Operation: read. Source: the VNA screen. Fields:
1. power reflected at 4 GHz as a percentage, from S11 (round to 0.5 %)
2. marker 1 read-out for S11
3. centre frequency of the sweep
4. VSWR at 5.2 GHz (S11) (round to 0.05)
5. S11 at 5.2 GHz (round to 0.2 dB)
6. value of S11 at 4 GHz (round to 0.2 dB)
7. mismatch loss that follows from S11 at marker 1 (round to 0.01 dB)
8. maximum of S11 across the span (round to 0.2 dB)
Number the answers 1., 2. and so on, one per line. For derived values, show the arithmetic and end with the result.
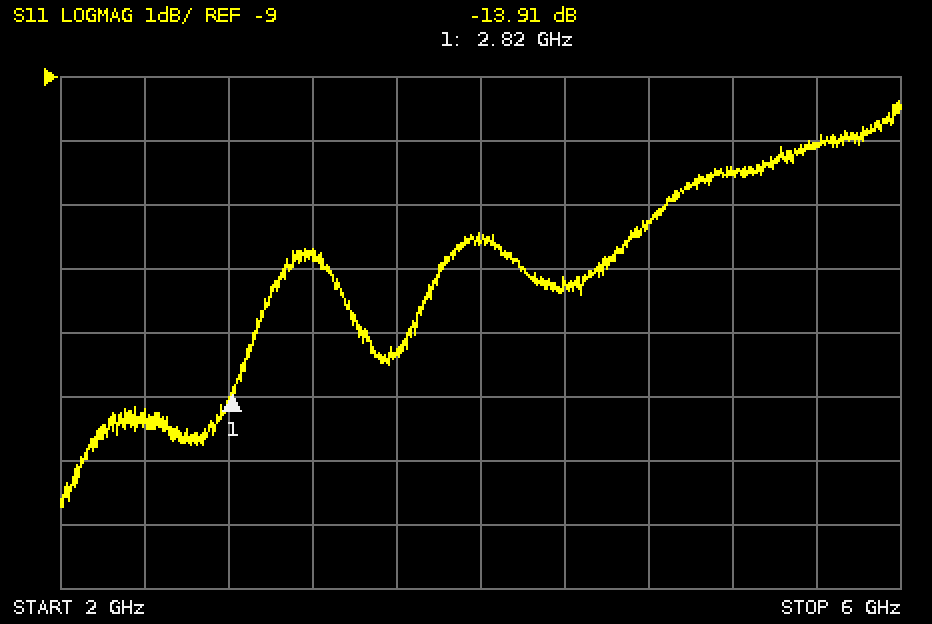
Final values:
1. 10^(-11.6/10) ≈ 6.92 %, so 7.0 % to the nearest 0.5 %
2. -13.91 dB
3. 4 GHz
4. |Γ| = 10^(-10.4/20) = 0.3020; VSWR = (1 + 0.3020)/(1 − 0.3020) ≈ 1.87, so 1.85 to the nearest 0.05
5. -10.4 dB
6. -11.6 dB
7. −10 log10(1 − 10^(-13.91/10)) ≈ 0.18 dB
8. -9.4 dB
